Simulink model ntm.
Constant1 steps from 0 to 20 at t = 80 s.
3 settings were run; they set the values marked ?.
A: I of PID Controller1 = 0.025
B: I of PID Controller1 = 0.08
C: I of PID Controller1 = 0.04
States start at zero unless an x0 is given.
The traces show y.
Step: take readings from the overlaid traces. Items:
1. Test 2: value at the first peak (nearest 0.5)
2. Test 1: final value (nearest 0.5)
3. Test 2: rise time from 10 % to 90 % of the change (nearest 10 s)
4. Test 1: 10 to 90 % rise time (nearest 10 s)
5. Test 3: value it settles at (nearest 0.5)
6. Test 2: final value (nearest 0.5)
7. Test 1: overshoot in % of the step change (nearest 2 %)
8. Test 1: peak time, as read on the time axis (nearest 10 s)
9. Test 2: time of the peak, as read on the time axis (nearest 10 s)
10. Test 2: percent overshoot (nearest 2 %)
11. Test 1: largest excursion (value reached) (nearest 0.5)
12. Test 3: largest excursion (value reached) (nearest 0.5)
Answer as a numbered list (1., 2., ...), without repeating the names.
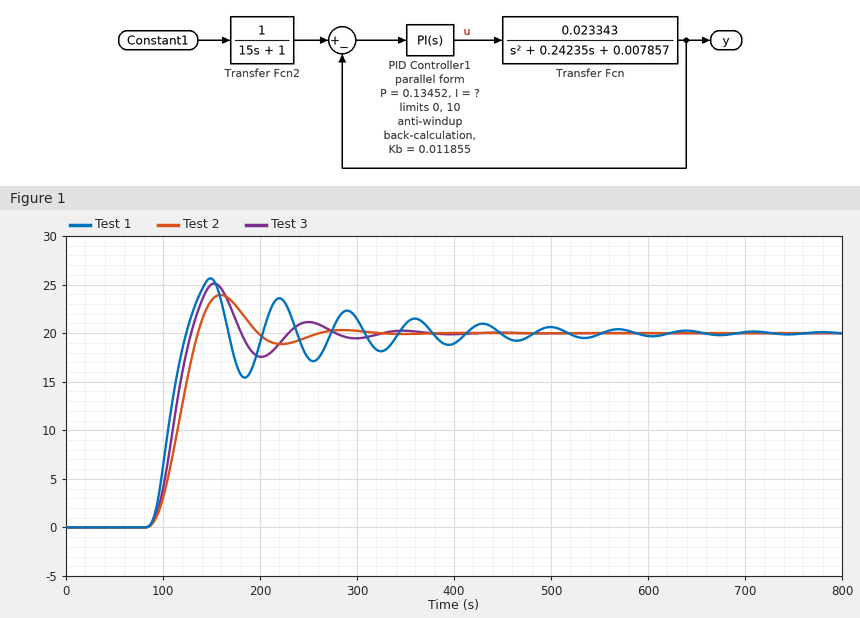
1. 24.0
2. 20.0
3. 30 s
4. 30 s
5. 20.0
6. 20.0
7. 28 %
8. 150 s
9. 160 s
10. 20 %
11. 25.5
12. 25.0
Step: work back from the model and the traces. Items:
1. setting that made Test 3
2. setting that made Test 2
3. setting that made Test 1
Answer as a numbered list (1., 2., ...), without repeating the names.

1. C
2. A
3. B
